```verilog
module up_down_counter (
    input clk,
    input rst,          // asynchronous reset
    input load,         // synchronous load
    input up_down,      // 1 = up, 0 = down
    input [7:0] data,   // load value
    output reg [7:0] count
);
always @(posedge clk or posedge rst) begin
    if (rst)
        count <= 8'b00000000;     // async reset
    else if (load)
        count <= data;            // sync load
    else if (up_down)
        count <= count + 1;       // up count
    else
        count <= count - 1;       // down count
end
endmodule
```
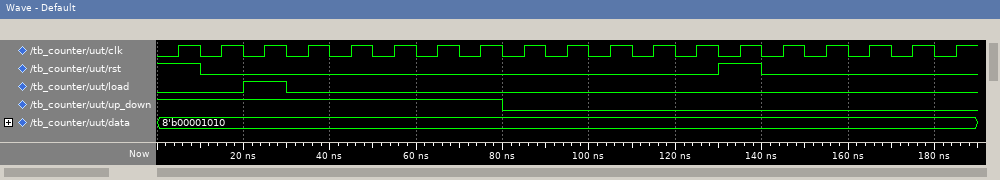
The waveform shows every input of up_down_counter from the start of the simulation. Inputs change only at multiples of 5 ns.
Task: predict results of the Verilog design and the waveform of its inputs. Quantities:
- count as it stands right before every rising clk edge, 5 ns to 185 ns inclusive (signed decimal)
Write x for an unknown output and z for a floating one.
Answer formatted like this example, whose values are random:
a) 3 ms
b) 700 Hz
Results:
a) 0, 0, 1, 10, 11, 12, 13, 14, 15, 14, 13, 12, 11, 0, 0, -1, -2, -3, -4
